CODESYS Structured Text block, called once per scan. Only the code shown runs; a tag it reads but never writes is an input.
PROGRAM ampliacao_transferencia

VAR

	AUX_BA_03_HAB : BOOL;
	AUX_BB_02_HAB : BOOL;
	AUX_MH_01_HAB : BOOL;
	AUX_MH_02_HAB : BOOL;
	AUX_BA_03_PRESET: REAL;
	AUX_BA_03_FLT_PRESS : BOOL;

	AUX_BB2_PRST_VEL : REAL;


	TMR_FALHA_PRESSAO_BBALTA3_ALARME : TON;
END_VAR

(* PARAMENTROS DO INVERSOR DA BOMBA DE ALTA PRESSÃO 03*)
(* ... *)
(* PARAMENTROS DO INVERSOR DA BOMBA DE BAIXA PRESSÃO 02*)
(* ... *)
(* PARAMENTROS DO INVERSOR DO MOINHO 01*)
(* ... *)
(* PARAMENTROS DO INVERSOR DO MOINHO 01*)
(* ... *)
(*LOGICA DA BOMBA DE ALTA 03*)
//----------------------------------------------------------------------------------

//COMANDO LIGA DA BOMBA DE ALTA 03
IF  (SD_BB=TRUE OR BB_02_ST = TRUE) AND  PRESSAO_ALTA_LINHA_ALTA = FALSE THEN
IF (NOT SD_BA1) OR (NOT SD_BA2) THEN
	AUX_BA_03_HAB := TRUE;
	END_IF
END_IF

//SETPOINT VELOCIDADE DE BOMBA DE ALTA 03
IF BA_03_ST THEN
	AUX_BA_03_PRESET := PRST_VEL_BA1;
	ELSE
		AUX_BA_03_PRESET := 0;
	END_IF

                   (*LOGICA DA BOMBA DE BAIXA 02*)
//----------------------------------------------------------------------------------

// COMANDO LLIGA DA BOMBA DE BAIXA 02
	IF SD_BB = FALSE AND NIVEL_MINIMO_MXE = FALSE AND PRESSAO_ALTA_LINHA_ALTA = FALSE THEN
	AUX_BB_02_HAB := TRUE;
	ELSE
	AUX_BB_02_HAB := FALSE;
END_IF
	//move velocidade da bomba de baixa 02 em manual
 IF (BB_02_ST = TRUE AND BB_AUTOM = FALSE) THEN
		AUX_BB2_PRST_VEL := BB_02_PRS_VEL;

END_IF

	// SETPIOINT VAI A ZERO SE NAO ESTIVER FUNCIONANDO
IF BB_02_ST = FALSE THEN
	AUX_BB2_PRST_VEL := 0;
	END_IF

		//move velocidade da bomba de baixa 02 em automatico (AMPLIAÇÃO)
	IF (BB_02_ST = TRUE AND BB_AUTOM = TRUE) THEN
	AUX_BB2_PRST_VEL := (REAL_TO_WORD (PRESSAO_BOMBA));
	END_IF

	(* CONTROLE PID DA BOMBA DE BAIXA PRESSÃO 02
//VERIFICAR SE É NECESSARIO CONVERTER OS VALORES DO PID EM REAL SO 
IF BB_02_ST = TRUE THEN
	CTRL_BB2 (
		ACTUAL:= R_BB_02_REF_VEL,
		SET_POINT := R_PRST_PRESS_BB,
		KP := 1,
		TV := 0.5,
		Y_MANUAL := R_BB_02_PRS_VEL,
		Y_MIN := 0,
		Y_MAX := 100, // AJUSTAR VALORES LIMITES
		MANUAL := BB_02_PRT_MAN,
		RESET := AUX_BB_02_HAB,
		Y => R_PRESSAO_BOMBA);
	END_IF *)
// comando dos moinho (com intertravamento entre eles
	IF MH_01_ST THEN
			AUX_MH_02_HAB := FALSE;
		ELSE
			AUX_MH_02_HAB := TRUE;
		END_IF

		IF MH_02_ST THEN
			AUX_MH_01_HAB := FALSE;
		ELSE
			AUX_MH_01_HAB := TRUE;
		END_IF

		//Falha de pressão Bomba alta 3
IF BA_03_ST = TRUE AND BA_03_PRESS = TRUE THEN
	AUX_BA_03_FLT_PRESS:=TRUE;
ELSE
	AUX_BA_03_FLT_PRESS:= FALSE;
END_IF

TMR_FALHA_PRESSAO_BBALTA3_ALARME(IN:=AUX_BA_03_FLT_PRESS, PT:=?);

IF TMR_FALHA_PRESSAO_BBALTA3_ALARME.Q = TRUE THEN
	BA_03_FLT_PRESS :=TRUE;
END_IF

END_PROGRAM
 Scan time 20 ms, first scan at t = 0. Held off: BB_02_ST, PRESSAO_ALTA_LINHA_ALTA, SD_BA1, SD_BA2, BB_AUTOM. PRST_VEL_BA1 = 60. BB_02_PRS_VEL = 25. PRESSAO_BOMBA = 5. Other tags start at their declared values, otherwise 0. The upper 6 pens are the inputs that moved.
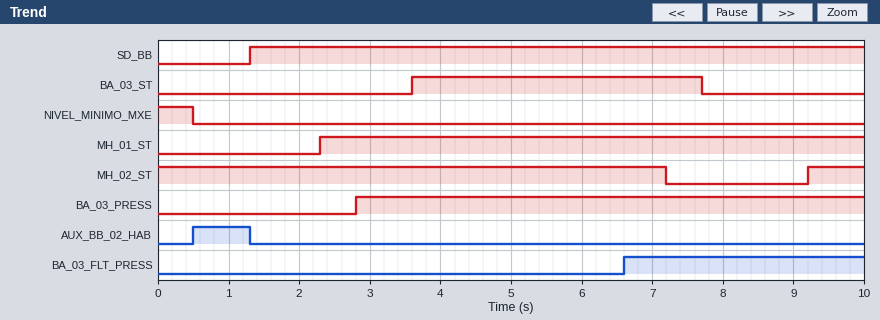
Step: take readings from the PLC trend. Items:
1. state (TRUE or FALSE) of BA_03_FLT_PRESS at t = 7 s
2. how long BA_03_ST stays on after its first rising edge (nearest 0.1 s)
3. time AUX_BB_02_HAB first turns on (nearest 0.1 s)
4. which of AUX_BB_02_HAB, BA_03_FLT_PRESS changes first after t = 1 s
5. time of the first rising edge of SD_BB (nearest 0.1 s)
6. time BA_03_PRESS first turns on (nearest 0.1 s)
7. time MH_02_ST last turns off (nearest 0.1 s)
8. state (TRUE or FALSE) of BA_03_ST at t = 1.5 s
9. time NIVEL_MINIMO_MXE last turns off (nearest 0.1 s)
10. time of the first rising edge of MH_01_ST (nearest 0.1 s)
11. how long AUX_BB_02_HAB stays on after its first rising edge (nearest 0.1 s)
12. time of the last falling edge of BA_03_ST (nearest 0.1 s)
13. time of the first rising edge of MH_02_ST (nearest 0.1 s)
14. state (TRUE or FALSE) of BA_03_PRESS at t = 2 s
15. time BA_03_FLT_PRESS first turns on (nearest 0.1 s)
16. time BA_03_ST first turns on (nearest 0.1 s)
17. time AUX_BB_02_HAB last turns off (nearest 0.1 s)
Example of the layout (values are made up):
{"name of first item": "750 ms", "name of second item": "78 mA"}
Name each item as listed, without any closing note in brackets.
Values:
{"state (TRUE or FALSE) of BA_03_FLT_PRESS at t = 7 s": "TRUE", "how long BA_03_ST stays on after its first rising edge": "4.1 s", "time AUX_BB_02_HAB first turns on": "0.5 s", "which of AUX_BB_02_HAB, BA_03_FLT_PRESS changes first after t = 1 s": "AUX_BB_02_HAB", "time of the first rising edge of SD_BB": "1.3 s", "time BA_03_PRESS first turns on": "2.8 s", "time MH_02_ST last turns off": "7.2 s", "state (TRUE or FALSE) of BA_03_ST at t = 1.5 s": "FALSE", "time NIVEL_MINIMO_MXE last turns off": "0.5 s", "time of the first rising edge of MH_01_ST": "2.3 s", "how long AUX_BB_02_HAB stays on after its first rising edge": "0.8 s", "time of the last falling edge of BA_03_ST": "7.7 s", "time of the first rising edge of MH_02_ST": "9.2 s", "state (TRUE or FALSE) of BA_03_PRESS at t = 2 s": "FALSE", "time BA_03_FLT_PRESS first turns on": "6.6 s", "time BA_03_ST first turns on": "3.6 s", "time AUX_BB_02_HAB last turns off": "1.3 s"}
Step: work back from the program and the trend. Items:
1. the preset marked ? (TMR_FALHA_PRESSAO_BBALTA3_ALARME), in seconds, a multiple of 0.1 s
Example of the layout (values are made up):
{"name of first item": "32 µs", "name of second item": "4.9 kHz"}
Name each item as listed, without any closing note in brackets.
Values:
{"the preset marked ? (TMR_FALHA_PRESSAO_BBALTA3_ALARME), in seconds, a multiple of 0.1 s": "3.0 s"}
